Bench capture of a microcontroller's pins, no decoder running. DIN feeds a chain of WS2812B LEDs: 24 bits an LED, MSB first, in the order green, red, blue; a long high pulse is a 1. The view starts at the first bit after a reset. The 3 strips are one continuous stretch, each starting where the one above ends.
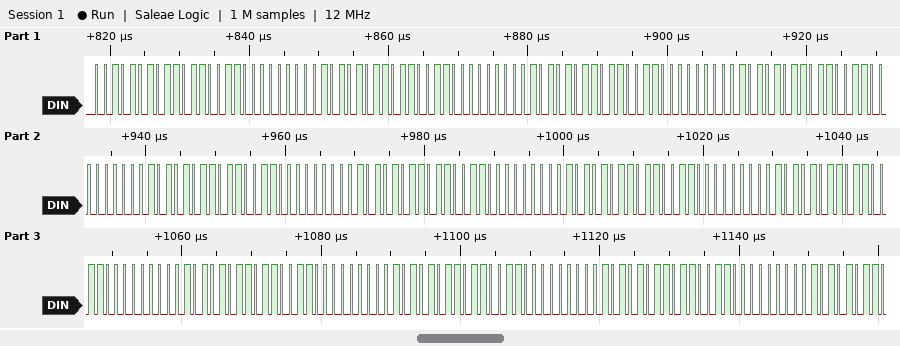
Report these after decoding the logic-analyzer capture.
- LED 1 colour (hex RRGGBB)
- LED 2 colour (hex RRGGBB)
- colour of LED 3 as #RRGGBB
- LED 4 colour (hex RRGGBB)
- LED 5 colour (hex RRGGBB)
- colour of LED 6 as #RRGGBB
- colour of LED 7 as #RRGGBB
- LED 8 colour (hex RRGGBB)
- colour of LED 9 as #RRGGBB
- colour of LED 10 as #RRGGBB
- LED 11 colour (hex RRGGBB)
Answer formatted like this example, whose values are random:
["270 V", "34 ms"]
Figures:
["#D92A80", "#D92A80", "#D92A80", "#D92A80", "#D92A80", "#D92A80", "#D92A80", "#D92A80", "#D92A80", "#D92A80", "#D92A80"]
